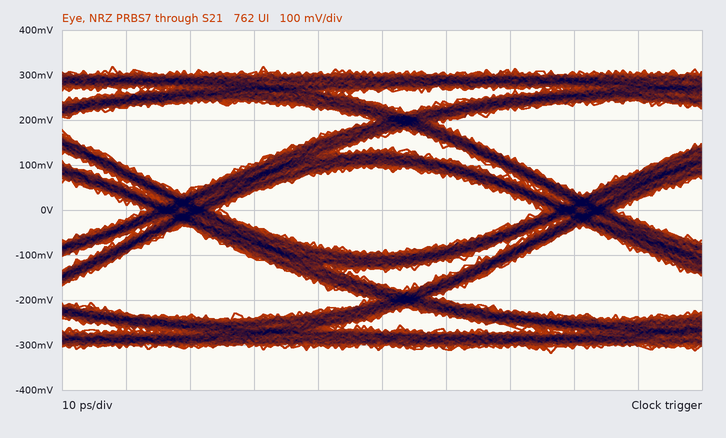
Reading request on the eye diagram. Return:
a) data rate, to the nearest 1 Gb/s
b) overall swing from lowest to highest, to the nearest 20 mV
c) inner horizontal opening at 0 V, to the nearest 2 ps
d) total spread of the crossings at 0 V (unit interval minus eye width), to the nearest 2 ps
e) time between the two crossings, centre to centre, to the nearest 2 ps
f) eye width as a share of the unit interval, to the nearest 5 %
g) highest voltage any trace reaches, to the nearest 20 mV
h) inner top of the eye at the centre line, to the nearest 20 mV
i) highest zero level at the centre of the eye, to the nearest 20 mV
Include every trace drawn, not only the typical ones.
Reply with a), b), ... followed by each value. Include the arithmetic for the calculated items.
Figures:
a) 16 Gb/s
b) 640 mV
c) 50 ps
d) 12 ps
e) 62 ps
f) 50 ps / 62 ps ≈ 80.6 %, so 80 % to the nearest 5 %
g) 320 mV
h) 100 mV
i) -100 mV
